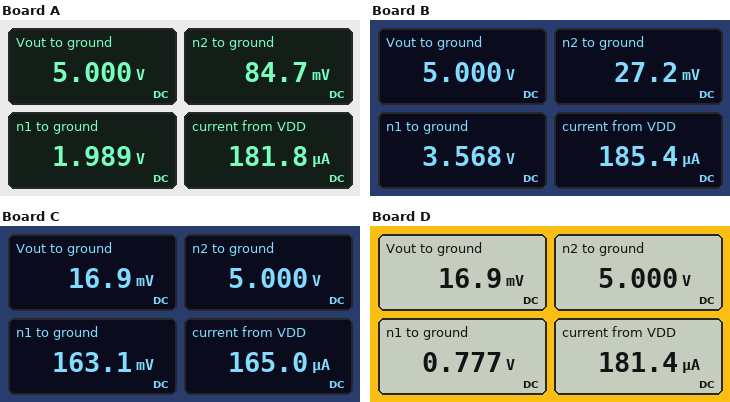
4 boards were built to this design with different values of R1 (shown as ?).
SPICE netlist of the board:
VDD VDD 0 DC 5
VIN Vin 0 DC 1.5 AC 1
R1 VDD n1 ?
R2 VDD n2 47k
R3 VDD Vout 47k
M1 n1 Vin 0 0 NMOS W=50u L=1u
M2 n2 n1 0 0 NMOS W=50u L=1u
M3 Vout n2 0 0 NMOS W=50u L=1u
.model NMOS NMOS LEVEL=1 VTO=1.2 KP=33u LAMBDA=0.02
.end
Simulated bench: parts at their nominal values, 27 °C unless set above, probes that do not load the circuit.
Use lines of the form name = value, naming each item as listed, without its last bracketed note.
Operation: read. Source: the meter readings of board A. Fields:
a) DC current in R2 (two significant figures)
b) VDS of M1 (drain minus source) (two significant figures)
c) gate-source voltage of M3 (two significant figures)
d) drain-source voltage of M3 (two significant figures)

DC current in R2 = 100 µA
VDS of M1 (drain minus source) = 2.0 V
gate-source voltage of M3 = 85 mV
drain-source voltage of M3 = 5.0 V
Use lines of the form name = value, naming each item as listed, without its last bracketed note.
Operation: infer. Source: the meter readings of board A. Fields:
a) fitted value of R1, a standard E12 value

fitted value of R1, a standard E12 value = 39 kΩ
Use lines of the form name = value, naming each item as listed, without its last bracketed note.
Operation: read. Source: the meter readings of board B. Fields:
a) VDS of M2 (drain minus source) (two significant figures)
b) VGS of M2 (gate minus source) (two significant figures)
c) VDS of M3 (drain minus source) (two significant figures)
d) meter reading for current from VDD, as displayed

VDS of M2 (drain minus source) = 27 mV
VGS of M2 (gate minus source) = 3.6 V
VDS of M3 (drain minus source) = 5.0 V
meter reading for current from VDD, as displayed = 185.4 µA
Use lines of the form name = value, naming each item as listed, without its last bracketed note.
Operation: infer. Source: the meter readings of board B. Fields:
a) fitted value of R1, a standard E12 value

fitted value of R1, a standard E12 value = 18 kΩ
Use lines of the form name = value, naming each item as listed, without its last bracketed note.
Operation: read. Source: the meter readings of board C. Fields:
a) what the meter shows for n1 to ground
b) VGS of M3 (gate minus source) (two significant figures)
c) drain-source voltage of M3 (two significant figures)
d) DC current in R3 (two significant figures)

what the meter shows for n1 to ground = 163.1 mV
VGS of M3 (gate minus source) = 5.0 V
drain-source voltage of M3 = 17 mV
DC current in R3 = 110 µA
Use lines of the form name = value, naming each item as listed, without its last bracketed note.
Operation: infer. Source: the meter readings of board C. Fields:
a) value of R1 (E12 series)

value of R1 = 82 kΩ
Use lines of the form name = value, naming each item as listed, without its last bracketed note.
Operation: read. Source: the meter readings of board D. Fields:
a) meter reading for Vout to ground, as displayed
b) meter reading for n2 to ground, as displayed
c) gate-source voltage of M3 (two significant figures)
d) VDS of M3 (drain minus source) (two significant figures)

meter reading for Vout to ground, as displayed = 16.9 mV
meter reading for n2 to ground, as displayed = 5.000 V
gate-source voltage of M3 = 5.0 V
VDS of M3 (drain minus source) = 17 mV
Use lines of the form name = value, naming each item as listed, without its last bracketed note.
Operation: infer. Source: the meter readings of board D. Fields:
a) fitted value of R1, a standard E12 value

fitted value of R1, a standard E12 value = 56 kΩ
